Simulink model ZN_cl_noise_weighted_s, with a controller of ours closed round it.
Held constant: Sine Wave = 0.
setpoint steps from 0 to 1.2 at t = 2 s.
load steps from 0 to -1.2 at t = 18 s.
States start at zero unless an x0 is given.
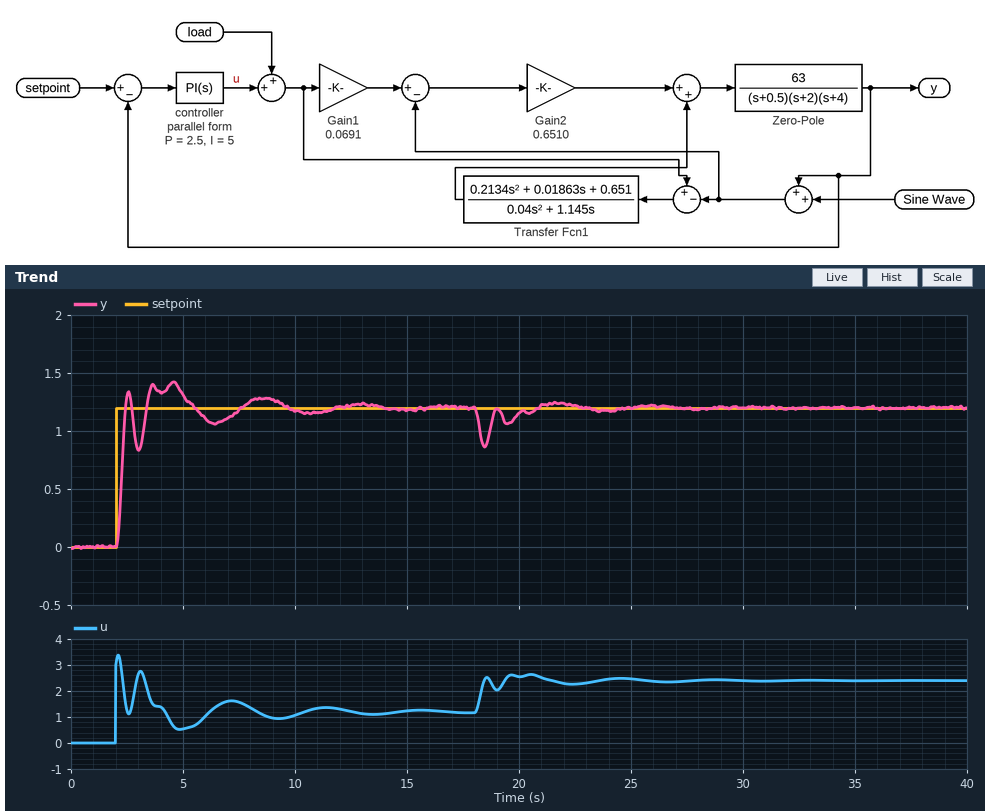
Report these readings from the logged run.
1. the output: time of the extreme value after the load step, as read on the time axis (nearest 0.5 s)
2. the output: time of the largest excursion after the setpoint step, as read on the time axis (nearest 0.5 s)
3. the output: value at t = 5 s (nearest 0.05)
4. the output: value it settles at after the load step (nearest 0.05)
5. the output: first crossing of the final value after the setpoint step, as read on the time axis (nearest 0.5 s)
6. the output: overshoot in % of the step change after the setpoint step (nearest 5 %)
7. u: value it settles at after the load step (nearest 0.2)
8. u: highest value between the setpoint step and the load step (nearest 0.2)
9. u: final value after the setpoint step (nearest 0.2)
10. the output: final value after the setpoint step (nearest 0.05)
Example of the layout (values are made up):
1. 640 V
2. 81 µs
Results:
1. 18.5 s
2. 4.5 s
3. 1.30
4. 1.20
5. 2.5 s
6. 20 %
7. 2.4
8. 3.4
9. 1.2
10. 1.20
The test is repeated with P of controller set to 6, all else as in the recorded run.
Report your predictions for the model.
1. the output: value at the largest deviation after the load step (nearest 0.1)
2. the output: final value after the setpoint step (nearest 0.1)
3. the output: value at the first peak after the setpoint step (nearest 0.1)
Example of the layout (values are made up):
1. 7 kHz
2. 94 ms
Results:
1. 1.0
2. 1.2
3. 1.6
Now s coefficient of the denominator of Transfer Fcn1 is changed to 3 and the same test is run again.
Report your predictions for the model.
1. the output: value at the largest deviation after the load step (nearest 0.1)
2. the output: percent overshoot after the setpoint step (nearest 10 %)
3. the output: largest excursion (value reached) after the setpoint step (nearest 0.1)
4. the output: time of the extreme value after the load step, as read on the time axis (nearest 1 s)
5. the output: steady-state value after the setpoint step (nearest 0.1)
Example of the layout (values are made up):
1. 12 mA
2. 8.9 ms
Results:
1. 1.0
2. 30 %
3. 1.6
4. 19 s
5. 1.2
